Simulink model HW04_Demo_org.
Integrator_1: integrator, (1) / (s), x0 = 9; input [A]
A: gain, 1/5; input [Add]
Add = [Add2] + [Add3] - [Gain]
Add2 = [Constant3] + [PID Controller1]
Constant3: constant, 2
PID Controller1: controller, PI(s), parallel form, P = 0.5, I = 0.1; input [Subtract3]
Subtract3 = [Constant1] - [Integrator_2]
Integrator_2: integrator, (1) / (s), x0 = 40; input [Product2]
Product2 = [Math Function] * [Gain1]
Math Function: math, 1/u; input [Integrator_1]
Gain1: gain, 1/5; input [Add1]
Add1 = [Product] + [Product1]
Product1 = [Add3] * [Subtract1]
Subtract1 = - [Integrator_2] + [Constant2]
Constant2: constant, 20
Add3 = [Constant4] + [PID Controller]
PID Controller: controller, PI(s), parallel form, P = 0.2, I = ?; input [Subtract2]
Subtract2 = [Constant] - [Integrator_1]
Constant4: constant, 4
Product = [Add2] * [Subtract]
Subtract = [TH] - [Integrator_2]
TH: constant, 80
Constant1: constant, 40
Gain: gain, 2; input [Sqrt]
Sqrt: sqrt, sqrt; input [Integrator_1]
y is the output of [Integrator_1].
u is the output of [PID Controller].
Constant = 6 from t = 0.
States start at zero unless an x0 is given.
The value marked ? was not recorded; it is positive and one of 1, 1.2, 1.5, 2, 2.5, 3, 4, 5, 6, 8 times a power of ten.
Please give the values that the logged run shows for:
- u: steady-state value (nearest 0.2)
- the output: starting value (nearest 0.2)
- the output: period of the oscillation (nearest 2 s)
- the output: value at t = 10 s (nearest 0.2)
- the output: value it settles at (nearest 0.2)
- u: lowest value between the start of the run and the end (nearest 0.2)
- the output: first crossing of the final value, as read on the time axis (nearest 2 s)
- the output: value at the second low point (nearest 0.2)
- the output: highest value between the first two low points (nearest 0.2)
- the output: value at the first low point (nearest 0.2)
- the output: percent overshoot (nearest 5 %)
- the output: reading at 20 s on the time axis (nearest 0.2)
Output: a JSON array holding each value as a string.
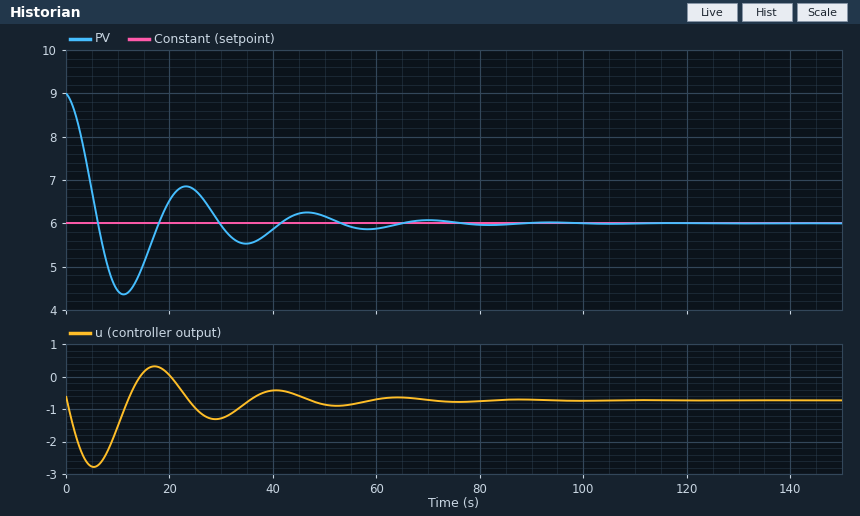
["-0.8", "9.0", "24 s", "4.4", "6.0", "-2.8", "6 s", "5.6", "6.8", "4.4", "55 %", "6.6"]
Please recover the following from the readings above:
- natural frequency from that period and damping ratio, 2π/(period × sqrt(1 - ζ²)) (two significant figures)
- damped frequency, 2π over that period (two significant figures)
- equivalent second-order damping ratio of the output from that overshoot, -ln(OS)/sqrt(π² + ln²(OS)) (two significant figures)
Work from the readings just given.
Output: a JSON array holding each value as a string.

["0.27 rad/s", "0.26 rad/s", "0.19"]
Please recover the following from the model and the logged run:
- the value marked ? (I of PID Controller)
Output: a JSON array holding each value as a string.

["0.25"]
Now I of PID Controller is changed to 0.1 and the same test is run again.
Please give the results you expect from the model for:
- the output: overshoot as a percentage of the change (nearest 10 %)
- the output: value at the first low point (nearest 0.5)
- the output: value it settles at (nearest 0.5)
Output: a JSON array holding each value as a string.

["30 %", "5.0", "6.0"]
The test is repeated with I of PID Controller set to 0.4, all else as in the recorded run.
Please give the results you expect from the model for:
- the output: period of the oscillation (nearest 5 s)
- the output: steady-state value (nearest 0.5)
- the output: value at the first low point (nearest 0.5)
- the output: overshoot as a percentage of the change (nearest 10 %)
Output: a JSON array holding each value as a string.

["20 s", "6.0", "4.0", "70 %"]
